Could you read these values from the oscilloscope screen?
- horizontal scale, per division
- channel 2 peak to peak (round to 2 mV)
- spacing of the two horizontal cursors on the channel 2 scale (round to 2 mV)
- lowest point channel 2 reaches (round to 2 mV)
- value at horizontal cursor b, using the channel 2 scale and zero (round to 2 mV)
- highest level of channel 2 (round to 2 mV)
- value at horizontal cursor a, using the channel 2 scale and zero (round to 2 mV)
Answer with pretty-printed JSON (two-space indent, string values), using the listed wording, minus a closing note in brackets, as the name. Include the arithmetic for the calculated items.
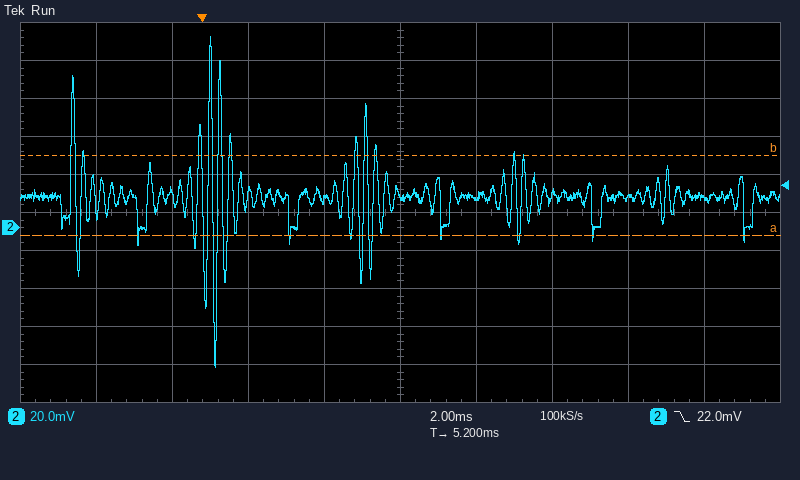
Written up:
{
  "horizontal scale, per division": "2 ms",
  "channel 2 peak to peak": "100 mV − (-74 mV) = 174 mV",
  "spacing of the two horizontal cursors on the channel 2 scale": "42 mV",
  "lowest point channel 2 reaches": "-74 mV",
  "value at horizontal cursor b, using the channel 2 scale and zero": "38 mV",
  "highest level of channel 2": "100 mV",
  "value at horizontal cursor a, using the channel 2 scale and zero": "-4 mV"
}
